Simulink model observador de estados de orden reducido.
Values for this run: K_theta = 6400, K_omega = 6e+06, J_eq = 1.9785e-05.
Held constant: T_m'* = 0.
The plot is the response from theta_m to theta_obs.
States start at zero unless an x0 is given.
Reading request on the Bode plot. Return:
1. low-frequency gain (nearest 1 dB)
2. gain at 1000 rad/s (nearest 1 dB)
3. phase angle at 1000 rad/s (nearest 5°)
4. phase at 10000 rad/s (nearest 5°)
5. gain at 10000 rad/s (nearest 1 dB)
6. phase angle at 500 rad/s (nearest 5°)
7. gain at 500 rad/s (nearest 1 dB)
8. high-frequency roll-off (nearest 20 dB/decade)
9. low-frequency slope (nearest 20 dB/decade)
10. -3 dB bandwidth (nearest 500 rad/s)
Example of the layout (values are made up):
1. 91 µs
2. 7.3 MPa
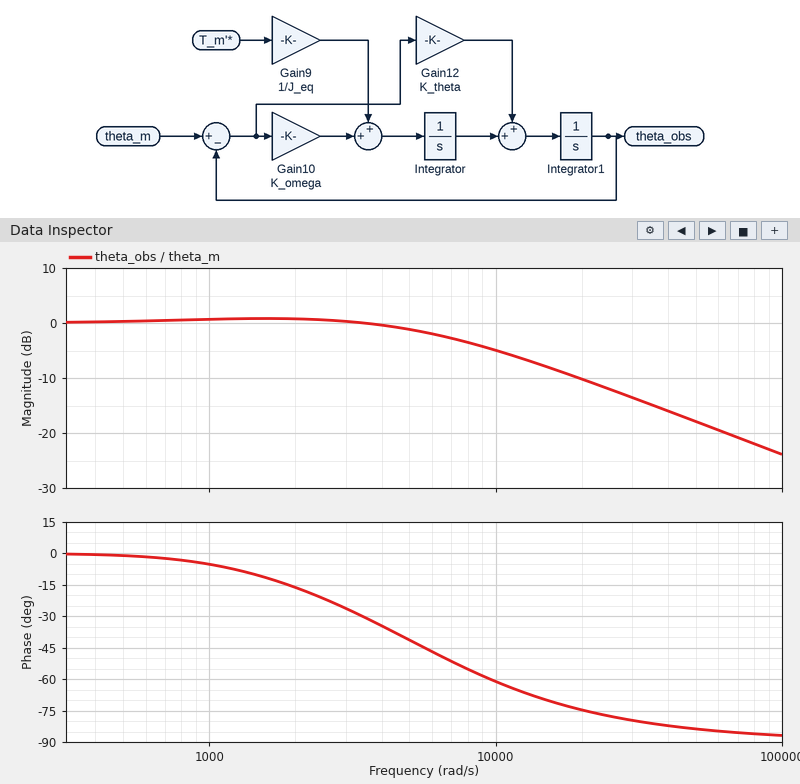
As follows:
1. 0 dB
2. 1 dB
3. -5°
4. -60°
5. -5 dB
6. 0°
7. 0 dB
8. -20 dB/decade
9. 0 dB/decade
10. 7000 rad/s
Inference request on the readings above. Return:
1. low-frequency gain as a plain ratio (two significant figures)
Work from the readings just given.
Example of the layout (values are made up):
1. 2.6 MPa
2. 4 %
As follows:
1. 1.0
